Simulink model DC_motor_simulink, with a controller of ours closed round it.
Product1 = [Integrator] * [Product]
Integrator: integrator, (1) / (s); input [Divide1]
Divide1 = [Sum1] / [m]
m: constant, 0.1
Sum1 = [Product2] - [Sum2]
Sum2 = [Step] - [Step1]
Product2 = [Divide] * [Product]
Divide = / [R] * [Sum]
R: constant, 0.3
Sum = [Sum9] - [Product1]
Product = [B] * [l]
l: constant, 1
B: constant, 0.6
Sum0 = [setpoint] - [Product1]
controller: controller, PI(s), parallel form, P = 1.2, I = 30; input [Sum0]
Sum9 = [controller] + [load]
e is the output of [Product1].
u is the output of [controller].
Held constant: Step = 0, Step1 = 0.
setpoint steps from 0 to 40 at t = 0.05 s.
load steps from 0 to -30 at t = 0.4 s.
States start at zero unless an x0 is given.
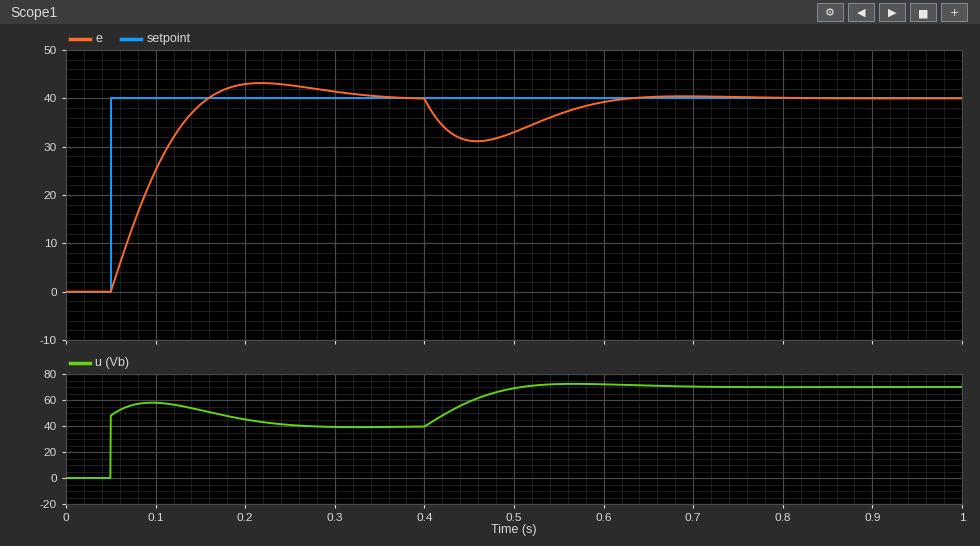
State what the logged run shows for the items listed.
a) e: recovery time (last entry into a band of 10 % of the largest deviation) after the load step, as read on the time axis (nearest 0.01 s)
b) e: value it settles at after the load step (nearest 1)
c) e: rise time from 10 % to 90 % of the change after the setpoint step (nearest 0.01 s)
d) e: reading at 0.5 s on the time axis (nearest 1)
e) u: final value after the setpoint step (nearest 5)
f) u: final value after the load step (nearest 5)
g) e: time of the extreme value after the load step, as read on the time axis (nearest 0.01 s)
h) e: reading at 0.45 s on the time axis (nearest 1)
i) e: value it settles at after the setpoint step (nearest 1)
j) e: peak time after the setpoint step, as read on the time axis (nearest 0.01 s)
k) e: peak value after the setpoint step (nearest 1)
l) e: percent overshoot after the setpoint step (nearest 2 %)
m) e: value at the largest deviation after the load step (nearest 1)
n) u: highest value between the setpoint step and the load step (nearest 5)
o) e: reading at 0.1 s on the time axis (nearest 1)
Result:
0.60 s
40
0.08 s
33
40
70
0.46 s
31
40
0.22 s
43
8 %
31
60
25
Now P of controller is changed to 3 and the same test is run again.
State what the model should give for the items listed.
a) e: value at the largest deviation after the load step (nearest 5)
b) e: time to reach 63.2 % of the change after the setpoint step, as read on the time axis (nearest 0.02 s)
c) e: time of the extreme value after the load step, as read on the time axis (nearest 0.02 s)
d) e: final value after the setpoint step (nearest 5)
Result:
35
0.08 s
0.44 s
40
